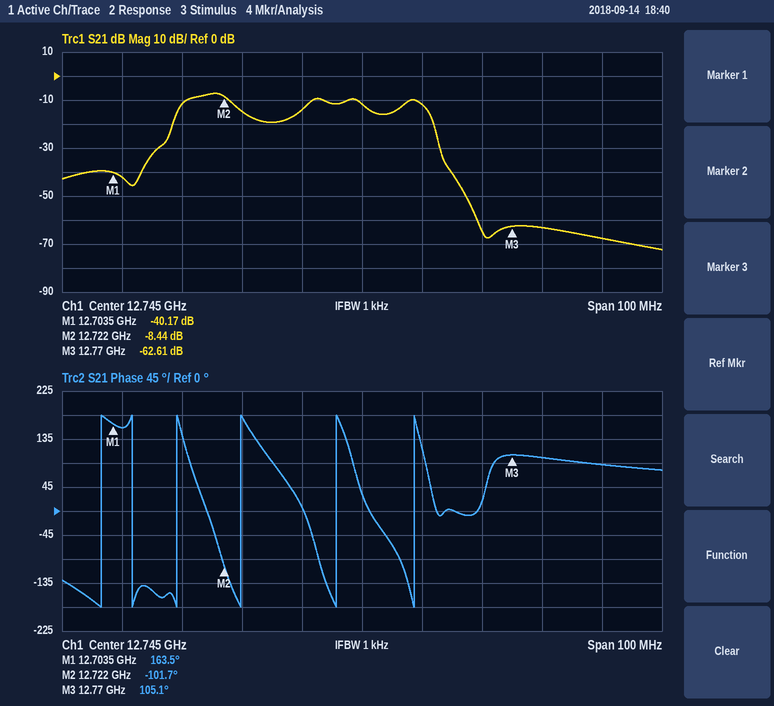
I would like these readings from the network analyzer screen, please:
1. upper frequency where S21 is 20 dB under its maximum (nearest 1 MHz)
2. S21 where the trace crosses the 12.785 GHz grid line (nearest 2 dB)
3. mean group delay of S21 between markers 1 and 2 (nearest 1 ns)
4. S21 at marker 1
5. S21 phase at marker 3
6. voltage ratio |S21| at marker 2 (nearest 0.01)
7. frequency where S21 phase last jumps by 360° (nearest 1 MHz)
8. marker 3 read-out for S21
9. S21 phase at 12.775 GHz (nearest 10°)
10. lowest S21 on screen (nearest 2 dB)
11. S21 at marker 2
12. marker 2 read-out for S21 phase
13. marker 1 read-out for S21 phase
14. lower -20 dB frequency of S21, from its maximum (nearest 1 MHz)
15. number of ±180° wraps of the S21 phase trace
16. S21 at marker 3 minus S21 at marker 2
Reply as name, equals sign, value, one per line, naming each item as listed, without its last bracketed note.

upper frequency where S21 is 20 dB under its maximum = 12.758 GHz
S21 where the trace crosses the 12.785 GHz grid line = -68 dB
mean group delay of S21 between markers 1 and 2 = 40 ns
S21 at marker 1 = -40.17 dB
S21 phase at marker 3 = 105.1°
voltage ratio |S21| at marker 2 = 0.38
frequency where S21 phase last jumps by 360° = 12.754 GHz
marker 3 read-out for S21 = -62.61 dB
S21 phase at 12.775 GHz = 100°
lowest S21 on screen = -72 dB
S21 at marker 2 = -8.44 dB
marker 2 read-out for S21 phase = -101.7°
marker 1 read-out for S21 phase = 163.5°
lower -20 dB frequency of S21, from its maximum = 12.712 GHz
number of ±180° wraps of the S21 phase trace = 6
S21 at marker 3 minus S21 at marker 2 = -54.17 dB
